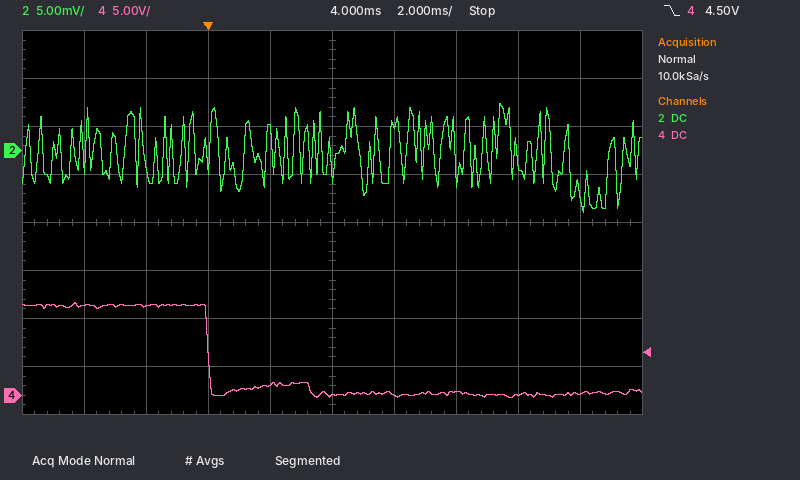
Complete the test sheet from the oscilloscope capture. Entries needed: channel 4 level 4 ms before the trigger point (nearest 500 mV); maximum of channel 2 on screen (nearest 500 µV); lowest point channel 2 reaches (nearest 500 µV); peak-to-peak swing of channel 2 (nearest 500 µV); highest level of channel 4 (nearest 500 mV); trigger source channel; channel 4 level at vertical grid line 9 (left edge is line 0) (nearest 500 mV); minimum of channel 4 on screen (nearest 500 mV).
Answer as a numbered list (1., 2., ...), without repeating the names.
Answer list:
1. 9.5 V
2. 5.0 mV
3. -6.5 mV
4. 11.5 mV
5. 9.5 V
6. channel 4
7. 0.0 V
8. 0.0 V
